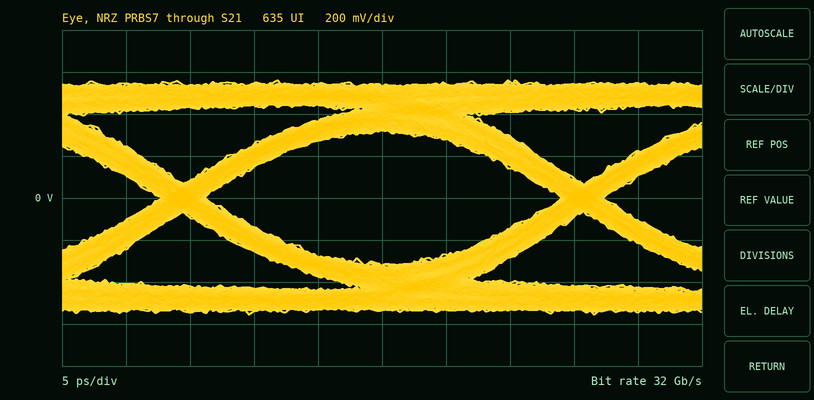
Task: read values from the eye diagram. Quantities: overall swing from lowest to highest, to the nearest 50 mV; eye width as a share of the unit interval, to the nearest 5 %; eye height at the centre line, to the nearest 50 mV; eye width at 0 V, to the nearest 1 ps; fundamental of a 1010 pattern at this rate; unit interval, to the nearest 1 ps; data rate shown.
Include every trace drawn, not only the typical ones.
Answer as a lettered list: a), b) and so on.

a) 1.10 V
b) 90 %
c) 650 mV
d) 28 ps
e) 16 GHz
f) 31 ps
g) 32 Gb/s
